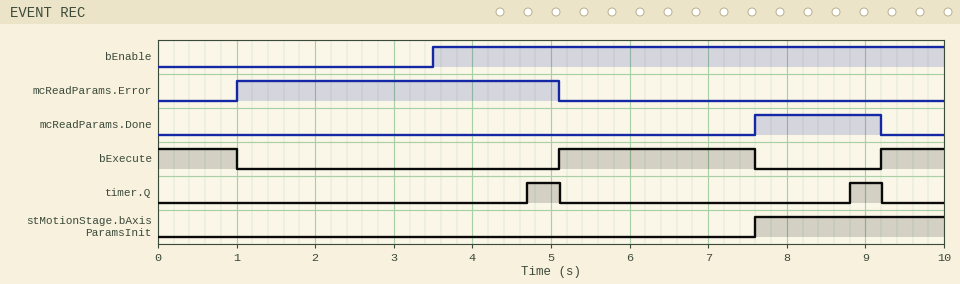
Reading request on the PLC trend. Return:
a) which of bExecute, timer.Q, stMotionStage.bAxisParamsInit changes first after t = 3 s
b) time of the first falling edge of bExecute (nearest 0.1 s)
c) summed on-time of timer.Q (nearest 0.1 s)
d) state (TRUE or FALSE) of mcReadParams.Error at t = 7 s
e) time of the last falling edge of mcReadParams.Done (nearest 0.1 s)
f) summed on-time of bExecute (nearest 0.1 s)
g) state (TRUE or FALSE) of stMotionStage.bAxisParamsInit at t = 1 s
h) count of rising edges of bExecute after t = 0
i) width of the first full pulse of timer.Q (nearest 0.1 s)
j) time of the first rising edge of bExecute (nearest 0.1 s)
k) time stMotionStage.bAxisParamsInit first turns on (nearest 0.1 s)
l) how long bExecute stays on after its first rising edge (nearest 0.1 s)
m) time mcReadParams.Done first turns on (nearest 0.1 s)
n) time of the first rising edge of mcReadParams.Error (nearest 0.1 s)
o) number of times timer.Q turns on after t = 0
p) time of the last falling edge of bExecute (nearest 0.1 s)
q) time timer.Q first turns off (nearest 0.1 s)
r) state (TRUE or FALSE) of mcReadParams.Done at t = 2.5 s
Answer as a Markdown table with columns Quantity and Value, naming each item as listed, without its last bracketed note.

| Quantity | Value |
|---|---|
| which of bExecute, timer.Q, stMotionStage.bAxisParamsInit changes first after t = 3 s | timer.Q |
| time of the first falling edge of bExecute | 1.0 s |
| summed on-time of timer.Q | 0.8 s |
| state (TRUE or FALSE) of mcReadParams.Error at t = 7 s | FALSE |
| time of the last falling edge of mcReadParams.Done | 9.2 s |
| summed on-time of bExecute | 4.3 s |
| state (TRUE or FALSE) of stMotionStage.bAxisParamsInit at t = 1 s | FALSE |
| count of rising edges of bExecute after t = 0 | 2 |
| width of the first full pulse of timer.Q | 0.4 s |
| time of the first rising edge of bExecute | 5.1 s |
| time stMotionStage.bAxisParamsInit first turns on | 7.6 s |
| how long bExecute stays on after its first rising edge | 2.5 s |
| time mcReadParams.Done first turns on | 7.6 s |
| time of the first rising edge of mcReadParams.Error | 1.0 s |
| number of times timer.Q turns on after t = 0 | 2 |
| time of the last falling edge of bExecute | 7.6 s |
| time timer.Q first turns off | 5.1 s |
| state (TRUE or FALSE) of mcReadParams.Done at t = 2.5 s | FALSE |
